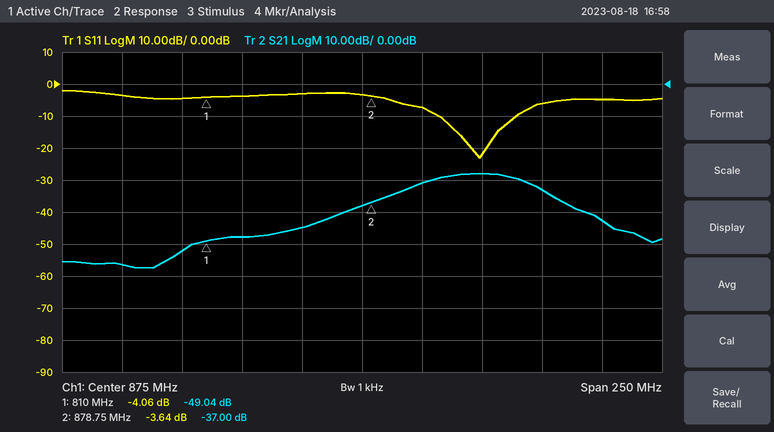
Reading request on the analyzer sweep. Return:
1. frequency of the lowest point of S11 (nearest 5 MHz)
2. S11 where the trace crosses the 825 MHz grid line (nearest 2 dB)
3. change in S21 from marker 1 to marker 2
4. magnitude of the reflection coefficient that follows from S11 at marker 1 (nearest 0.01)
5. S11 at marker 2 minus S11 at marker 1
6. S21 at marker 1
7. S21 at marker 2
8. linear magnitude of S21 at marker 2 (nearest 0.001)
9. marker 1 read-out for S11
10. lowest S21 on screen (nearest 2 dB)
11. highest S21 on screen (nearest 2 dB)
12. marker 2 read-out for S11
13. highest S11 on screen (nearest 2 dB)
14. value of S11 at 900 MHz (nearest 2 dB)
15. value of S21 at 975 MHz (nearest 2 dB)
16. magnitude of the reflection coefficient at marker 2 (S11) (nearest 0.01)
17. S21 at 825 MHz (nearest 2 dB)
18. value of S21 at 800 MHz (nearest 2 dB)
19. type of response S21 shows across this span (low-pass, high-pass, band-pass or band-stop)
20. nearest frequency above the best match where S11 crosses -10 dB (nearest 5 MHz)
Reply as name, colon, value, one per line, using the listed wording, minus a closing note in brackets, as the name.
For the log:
frequency of the lowest point of S11: 925 MHz
S11 where the trace crosses the 825 MHz grid line: -4 dB
change in S21 from marker 1 to marker 2: 12.04 dB
magnitude of the reflection coefficient that follows from S11 at marker 1: 0.63
S11 at marker 2 minus S11 at marker 1: 0.42 dB
S21 at marker 1: -49.04 dB
S21 at marker 2: -37.00 dB
linear magnitude of S21 at marker 2: 0.014
marker 1 read-out for S11: -4.06 dB
lowest S21 on screen: -58 dB
highest S21 on screen: -28 dB
marker 2 read-out for S11: -3.64 dB
highest S11 on screen: -2 dB
value of S11 at 900 MHz: -8 dB
value of S21 at 975 MHz: -42 dB
magnitude of the reflection coefficient at marker 2 (S11): 0.66
S21 at 825 MHz: -48 dB
value of S21 at 800 MHz: -52 dB
type of response S21 shows across this span: band-pass
nearest frequency above the best match where S11 crosses -10 dB: 940 MHz
